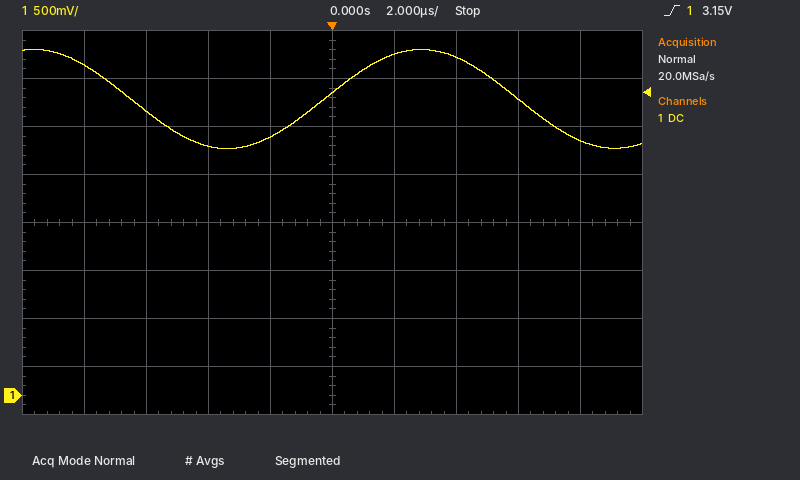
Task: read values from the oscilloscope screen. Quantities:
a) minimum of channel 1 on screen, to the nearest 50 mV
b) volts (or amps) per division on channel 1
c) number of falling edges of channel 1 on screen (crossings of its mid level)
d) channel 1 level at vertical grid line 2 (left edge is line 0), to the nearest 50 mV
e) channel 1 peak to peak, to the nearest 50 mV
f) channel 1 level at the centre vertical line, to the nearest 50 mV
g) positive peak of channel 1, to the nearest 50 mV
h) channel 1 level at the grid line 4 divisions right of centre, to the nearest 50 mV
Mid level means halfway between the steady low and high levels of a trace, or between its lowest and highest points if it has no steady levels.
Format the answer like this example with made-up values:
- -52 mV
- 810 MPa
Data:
- 2.55 V
- 500 mV
- 2
- 2.95 V
- 1.05 V
- 3.15 V
- 3.60 V
- 2.65 V
